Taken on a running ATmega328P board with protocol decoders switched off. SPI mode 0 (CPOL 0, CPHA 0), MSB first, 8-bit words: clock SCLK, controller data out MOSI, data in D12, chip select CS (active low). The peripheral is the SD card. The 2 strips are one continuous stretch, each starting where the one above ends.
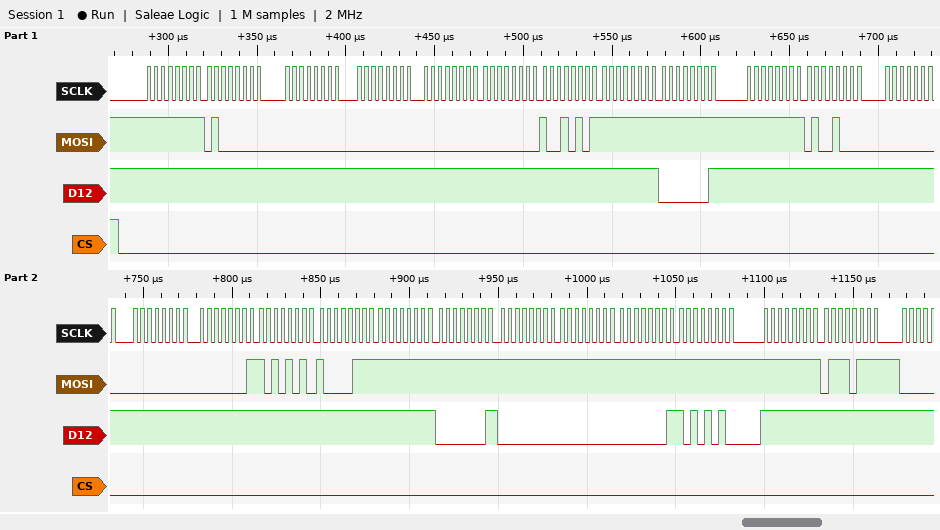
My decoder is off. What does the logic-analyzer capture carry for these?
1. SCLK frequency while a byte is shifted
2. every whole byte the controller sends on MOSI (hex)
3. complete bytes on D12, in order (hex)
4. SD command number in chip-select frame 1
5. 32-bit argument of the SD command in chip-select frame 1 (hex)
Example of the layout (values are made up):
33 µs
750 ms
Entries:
250 kHz
0xFF 0x40 0x00 0x00 0x00 0x00 0x95 0xFF 0xFF 0xFF 0x48 0x00 0x00 0x01 0xAA 0x87 0xFF 0xFF 0xFF 0xFF 0xFF 0xFF 0xFF 0x77
0xFF 0xFF 0xFF 0xFF 0xFF 0xFF 0xFF 0xFF 0x01 0xFF 0xFF 0xFF 0xFF 0xFF 0xFF 0xFF 0xFF 0x01 0x00 0x00 0x01 0xAA 0xFF 0xFF
CMD0
0x00000000
